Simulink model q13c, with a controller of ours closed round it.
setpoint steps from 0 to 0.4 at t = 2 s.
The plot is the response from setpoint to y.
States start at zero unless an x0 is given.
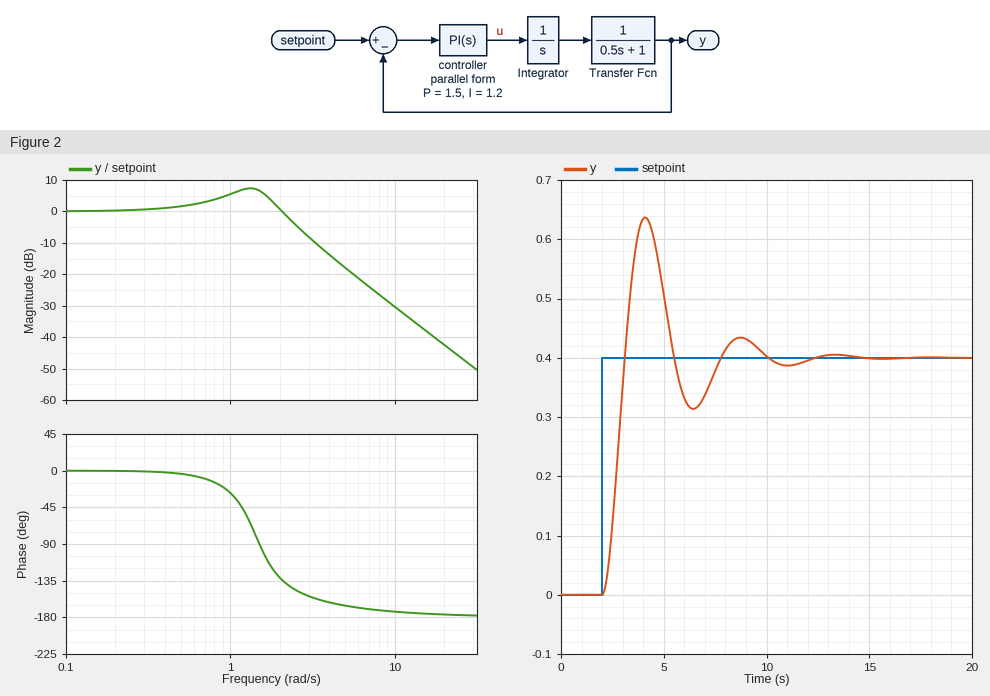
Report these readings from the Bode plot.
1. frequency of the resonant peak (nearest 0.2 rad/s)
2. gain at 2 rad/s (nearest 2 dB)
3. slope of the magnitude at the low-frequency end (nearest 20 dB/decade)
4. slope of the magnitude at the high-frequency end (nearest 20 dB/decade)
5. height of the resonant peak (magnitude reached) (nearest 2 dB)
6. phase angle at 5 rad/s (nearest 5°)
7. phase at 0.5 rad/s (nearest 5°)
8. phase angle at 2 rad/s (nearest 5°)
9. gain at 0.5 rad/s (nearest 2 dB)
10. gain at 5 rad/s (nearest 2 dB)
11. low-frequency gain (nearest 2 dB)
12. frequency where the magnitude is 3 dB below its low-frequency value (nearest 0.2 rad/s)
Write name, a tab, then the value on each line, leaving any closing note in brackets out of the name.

frequency of the resonant peak	1.4 rad/s
gain at 2 rad/s	0 dB
slope of the magnitude at the low-frequency end	0 dB/decade
slope of the magnitude at the high-frequency end	-40 dB/decade
height of the resonant peak (magnitude reached)	8 dB
phase angle at 5 rad/s	-165°
phase at 0.5 rad/s	-5°
phase angle at 2 rad/s	-130°
gain at 0.5 rad/s	2 dB
gain at 5 rad/s	-18 dB
low-frequency gain	0 dB
frequency where the magnitude is 3 dB below its low-frequency value	2.4 rad/s
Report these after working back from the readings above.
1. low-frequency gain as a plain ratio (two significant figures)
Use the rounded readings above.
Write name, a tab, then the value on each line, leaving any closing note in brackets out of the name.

low-frequency gain as a plain ratio	1.0
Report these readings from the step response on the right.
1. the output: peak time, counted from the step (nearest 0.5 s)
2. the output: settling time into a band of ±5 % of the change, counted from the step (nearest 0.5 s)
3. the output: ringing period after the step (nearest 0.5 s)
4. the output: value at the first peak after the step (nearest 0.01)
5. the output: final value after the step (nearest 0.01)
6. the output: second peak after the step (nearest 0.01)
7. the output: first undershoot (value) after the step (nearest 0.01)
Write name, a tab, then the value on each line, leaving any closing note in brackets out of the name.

the output: peak time, counted from the step	2.0 s
the output: settling time into a band of ±5 % of the change, counted from the step	7.5 s
the output: ringing period after the step	4.5 s
the output: value at the first peak after the step	0.64
the output: final value after the step	0.40
the output: second peak after the step	0.43
the output: first undershoot (value) after the step	0.31
